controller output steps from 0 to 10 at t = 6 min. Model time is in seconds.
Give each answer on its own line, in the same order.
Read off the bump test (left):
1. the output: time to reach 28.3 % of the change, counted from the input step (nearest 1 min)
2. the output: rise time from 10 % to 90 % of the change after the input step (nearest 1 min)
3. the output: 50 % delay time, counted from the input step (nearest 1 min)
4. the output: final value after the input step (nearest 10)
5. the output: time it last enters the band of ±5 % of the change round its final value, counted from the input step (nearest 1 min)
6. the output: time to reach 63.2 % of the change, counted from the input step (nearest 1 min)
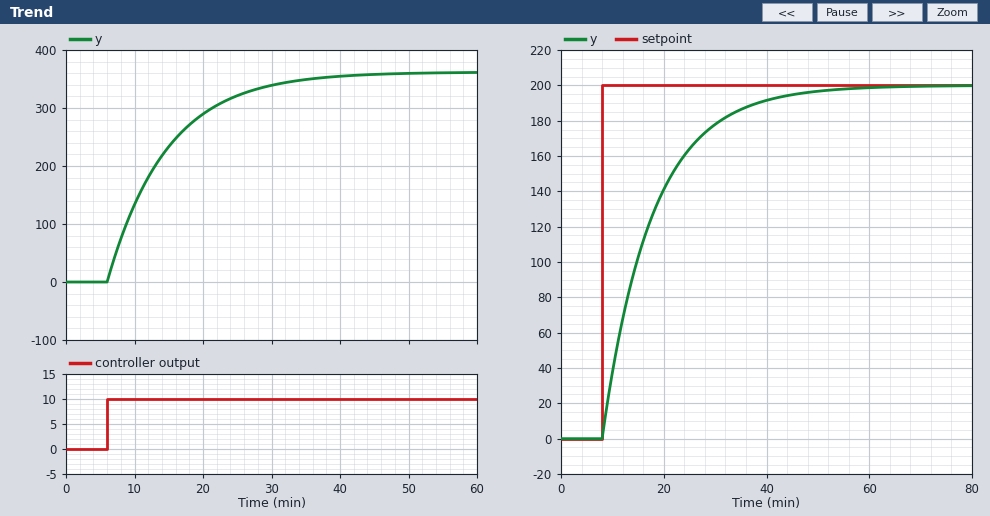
3 min
19 min
6 min
360
26 min
9 min
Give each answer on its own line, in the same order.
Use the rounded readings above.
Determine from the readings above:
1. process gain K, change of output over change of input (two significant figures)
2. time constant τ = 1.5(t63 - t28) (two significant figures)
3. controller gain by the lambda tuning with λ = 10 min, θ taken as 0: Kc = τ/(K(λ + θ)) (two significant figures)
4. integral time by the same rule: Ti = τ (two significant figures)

36
9.0 min
0.025
9.0 min
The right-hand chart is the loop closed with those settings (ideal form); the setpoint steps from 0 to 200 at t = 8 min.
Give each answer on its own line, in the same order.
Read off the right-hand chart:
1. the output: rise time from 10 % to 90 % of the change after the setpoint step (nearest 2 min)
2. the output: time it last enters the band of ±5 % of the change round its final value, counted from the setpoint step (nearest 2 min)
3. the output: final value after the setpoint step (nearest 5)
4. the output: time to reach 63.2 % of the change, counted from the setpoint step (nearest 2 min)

22 min
30 min
200
10 min
